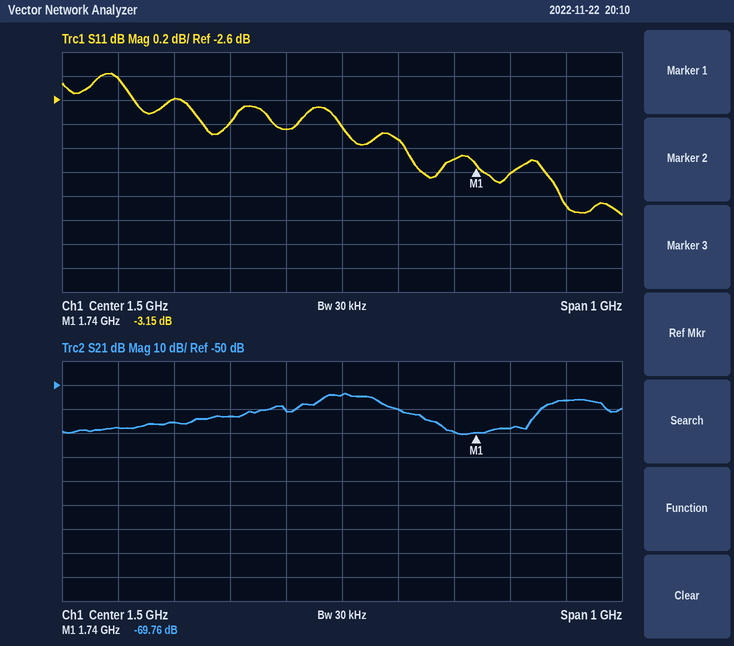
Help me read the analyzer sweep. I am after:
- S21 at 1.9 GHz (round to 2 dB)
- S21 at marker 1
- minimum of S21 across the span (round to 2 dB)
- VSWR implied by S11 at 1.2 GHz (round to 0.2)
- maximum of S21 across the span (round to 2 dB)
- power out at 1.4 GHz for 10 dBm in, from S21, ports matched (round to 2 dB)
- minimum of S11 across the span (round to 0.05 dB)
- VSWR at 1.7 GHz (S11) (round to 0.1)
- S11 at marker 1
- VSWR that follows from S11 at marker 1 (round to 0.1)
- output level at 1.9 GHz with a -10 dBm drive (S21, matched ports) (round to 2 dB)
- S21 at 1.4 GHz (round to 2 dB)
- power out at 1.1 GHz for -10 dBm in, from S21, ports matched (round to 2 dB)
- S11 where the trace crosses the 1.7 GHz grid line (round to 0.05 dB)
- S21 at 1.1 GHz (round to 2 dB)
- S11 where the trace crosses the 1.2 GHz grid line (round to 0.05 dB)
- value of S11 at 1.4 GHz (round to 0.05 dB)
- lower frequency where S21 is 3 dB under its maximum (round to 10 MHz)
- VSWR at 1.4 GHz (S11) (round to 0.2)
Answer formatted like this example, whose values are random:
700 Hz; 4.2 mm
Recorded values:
-56 dB; -69.76 dB; -70 dB; 6.8; -54 dB; -50 dBm; -3.55 dB; 5.7; -3.15 dB; 5.6; -66 dBm; -60 dB; -78 dBm; -3.10 dB; -68 dB; -2.60 dB; -2.85 dB; 1.46 GHz; 6.2
